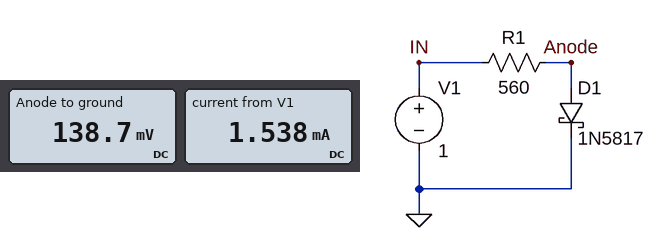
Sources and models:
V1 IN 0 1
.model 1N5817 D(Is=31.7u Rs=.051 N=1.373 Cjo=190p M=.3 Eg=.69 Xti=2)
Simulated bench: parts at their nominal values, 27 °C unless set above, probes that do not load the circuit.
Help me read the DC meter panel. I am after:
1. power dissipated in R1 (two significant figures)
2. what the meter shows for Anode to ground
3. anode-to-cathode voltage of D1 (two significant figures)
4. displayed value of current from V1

1.3 mW
138.7 mV
140 mV
1.538 mA
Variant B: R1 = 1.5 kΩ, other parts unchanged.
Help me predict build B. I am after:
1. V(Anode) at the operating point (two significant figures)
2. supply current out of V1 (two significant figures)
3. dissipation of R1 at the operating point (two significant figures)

110 mV
600 µA
530 µW
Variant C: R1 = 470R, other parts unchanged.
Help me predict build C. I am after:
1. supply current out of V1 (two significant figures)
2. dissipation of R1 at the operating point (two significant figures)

1.8 mA
1.6 mW
